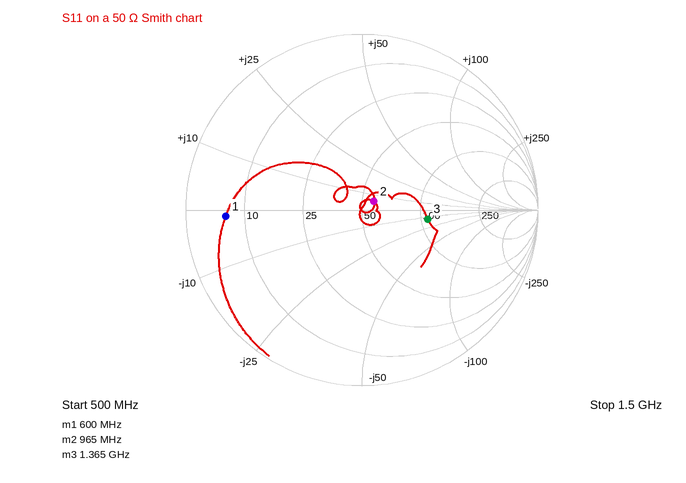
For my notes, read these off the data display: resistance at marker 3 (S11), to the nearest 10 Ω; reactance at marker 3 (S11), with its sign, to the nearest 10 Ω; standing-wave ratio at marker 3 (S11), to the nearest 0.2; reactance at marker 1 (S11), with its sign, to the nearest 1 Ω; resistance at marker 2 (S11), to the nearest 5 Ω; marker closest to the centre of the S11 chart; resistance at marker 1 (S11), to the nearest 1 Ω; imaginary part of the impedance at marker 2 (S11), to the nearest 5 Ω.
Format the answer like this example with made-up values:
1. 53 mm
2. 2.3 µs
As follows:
1. 110 Ω
2. -10 Ω
3. 2.2
4. -1 Ω
5. 55 Ω
6. marker 2
7. 6 Ω
8. +5 Ω
